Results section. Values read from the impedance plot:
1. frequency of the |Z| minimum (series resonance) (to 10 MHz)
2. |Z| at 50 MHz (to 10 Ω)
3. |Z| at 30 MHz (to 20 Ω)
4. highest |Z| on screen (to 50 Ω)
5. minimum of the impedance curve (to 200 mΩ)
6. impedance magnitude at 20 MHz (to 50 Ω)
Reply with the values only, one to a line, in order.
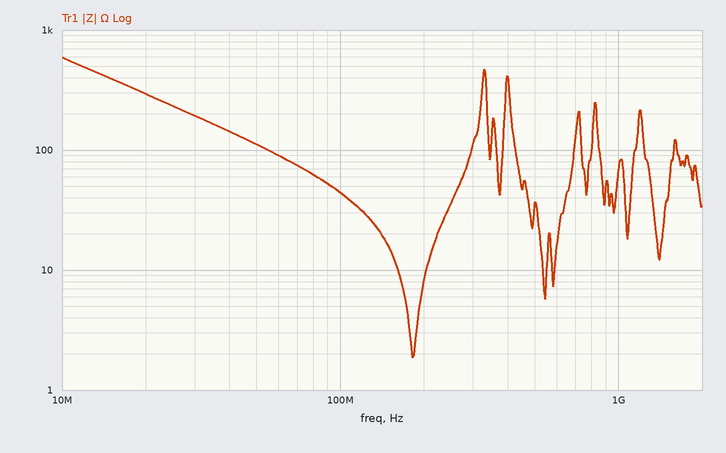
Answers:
180 MHz
110 Ω
200 Ω
600 Ω
1.8 Ω
300 Ω
